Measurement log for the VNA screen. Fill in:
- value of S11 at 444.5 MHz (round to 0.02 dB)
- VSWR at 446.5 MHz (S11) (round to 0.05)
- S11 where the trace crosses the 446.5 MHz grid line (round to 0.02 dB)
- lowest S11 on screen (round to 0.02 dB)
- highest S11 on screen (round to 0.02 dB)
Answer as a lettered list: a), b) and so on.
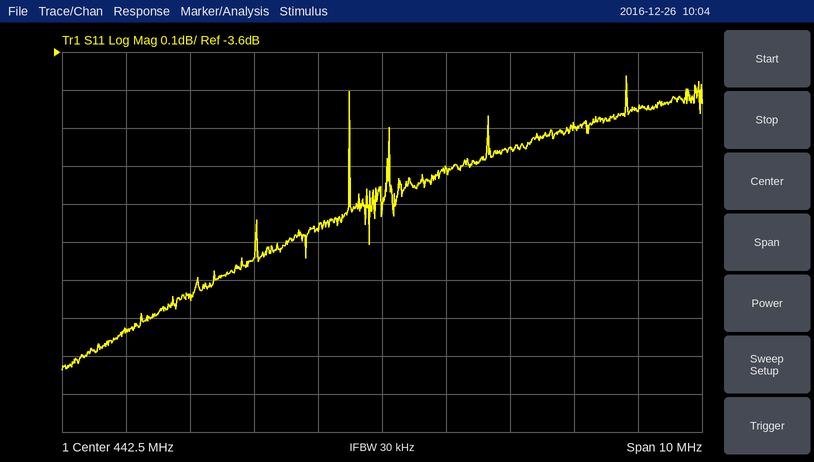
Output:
a) -3.86 dB
b) 4.70
c) -3.76 dB
d) -4.44 dB
e) -3.66 dB
